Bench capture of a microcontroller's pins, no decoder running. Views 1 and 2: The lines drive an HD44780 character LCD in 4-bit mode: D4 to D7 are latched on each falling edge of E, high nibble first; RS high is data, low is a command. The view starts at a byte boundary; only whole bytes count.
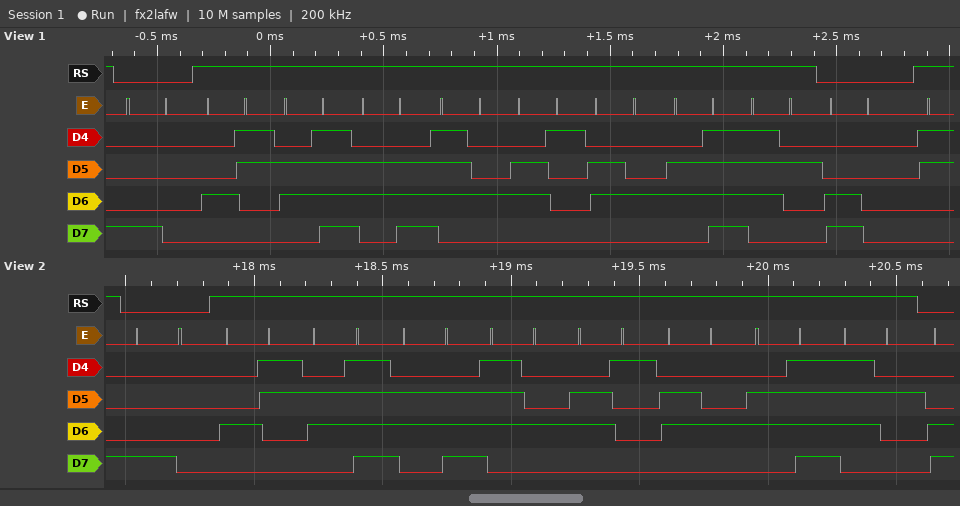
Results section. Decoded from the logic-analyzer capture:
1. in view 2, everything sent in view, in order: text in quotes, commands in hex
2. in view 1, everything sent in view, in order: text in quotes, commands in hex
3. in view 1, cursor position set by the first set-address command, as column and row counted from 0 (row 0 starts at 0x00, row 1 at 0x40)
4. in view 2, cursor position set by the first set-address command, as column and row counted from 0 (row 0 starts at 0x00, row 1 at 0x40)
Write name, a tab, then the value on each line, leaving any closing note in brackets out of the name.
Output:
in view 2, everything sent in view, in order: text in quotes, commands in hex	0x80 "Contador"
in view 1, everything sent in view, in order: text in quotes, commands in hex	0x80 "Contador" 0xC0
in view 1, cursor position set by the first set-address command, as column and row counted from 0	column 0, row 0
in view 2, cursor position set by the first set-address command, as column and row counted from 0	column 0, row 0
